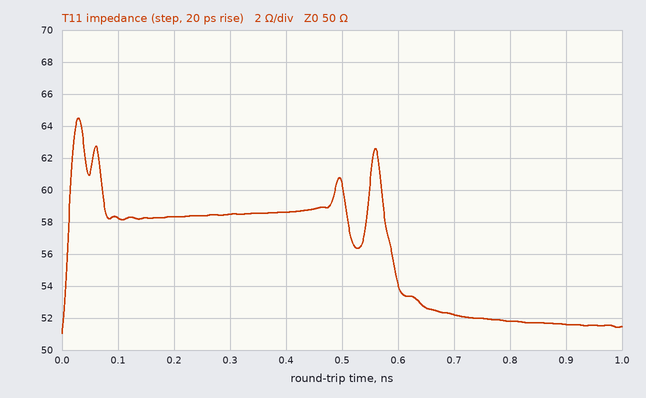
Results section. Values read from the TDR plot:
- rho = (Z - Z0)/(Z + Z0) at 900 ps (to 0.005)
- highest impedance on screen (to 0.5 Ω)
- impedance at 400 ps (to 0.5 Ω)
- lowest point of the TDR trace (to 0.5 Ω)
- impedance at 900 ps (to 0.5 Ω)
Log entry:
+0.015
64.5 Ω
58.5 Ω
51.0 Ω
51.5 Ω
